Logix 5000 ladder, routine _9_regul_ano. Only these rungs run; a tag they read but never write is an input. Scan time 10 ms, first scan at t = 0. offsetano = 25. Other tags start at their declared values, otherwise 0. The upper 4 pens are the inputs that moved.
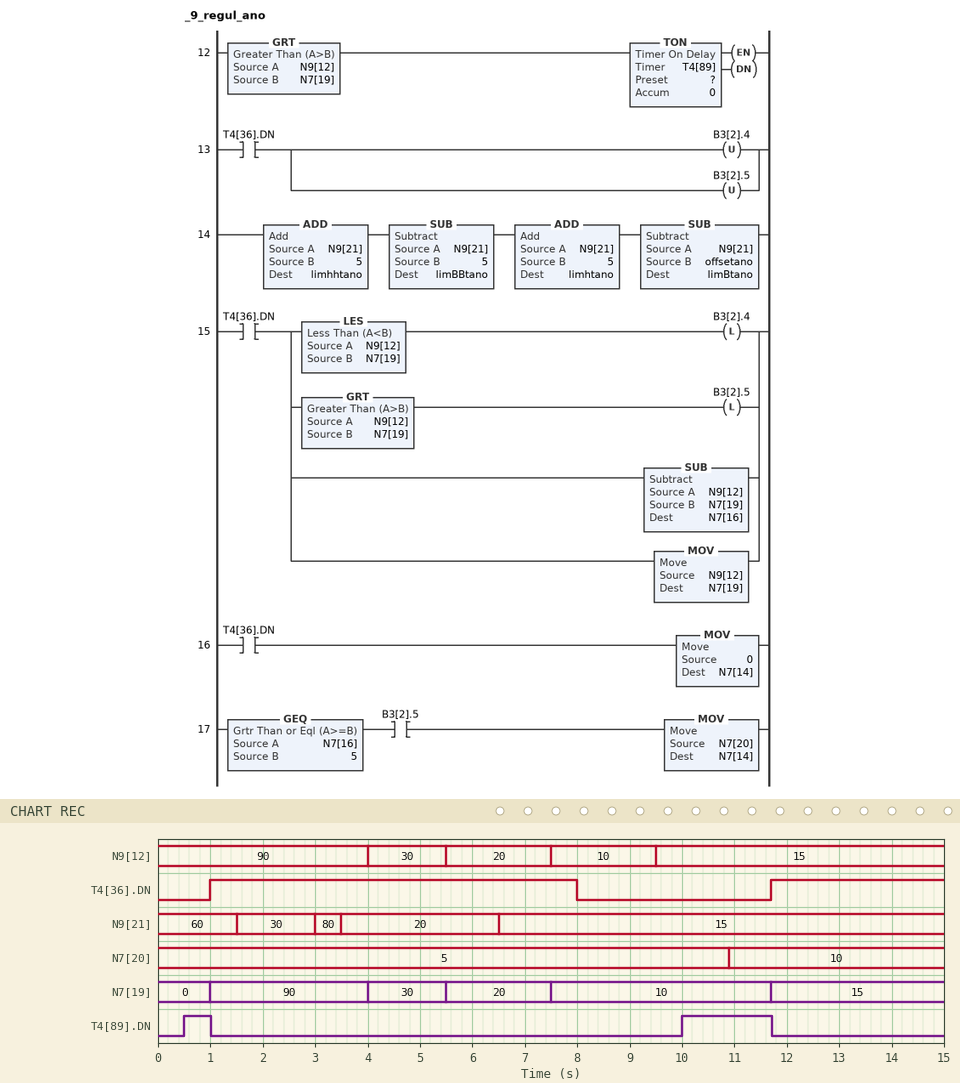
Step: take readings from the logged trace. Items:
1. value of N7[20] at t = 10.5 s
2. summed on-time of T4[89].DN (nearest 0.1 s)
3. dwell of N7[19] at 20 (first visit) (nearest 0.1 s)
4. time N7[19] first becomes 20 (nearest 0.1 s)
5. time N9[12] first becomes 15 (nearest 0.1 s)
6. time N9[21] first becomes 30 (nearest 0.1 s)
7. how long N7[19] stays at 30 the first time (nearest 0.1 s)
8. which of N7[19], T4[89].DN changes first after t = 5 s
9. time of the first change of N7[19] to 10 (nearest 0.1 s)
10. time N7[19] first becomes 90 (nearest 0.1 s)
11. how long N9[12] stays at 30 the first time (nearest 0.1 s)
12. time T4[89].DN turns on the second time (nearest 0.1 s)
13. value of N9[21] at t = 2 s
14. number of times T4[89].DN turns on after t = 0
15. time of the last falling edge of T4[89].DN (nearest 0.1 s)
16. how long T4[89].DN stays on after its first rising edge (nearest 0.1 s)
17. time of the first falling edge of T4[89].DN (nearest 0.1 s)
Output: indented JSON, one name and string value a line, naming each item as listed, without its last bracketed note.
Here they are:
{
  "value of N7[20] at t = 10.5 s": "5",
  "summed on-time of T4[89].DN": "2.2 s",
  "dwell of N7[19] at 20 (first visit)": "2.0 s",
  "time N7[19] first becomes 20": "5.5 s",
  "time N9[12] first becomes 15": "9.5 s",
  "time N9[21] first becomes 30": "1.5 s",
  "how long N7[19] stays at 30 the first time": "1.5 s",
  "which of N7[19], T4[89].DN changes first after t = 5 s": "N7[19]",
  "time of the first change of N7[19] to 10": "7.5 s",
  "time N7[19] first becomes 90": "1.0 s",
  "how long N9[12] stays at 30 the first time": "1.5 s",
  "time T4[89].DN turns on the second time": "10.0 s",
  "value of N9[21] at t = 2 s": "30",
  "number of times T4[89].DN turns on after t = 0": "2",
  "time of the last falling edge of T4[89].DN": "11.7 s",
  "how long T4[89].DN stays on after its first rising edge": "0.5 s",
  "time of the first falling edge of T4[89].DN": "1.0 s"
}
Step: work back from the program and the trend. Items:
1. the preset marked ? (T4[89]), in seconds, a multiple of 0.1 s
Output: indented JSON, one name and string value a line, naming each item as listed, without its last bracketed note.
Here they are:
{
  "the preset marked ? (T4[89]), in seconds, a multiple of 0.1 s": "0.5 s"
}
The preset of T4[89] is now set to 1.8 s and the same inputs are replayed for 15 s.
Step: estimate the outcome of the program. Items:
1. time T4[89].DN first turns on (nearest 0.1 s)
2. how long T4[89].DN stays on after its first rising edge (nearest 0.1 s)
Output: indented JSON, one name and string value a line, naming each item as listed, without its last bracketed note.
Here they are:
{
  "time T4[89].DN first turns on": "11.3 s",
  "how long T4[89].DN stays on after its first rising edge": "0.4 s"
}
